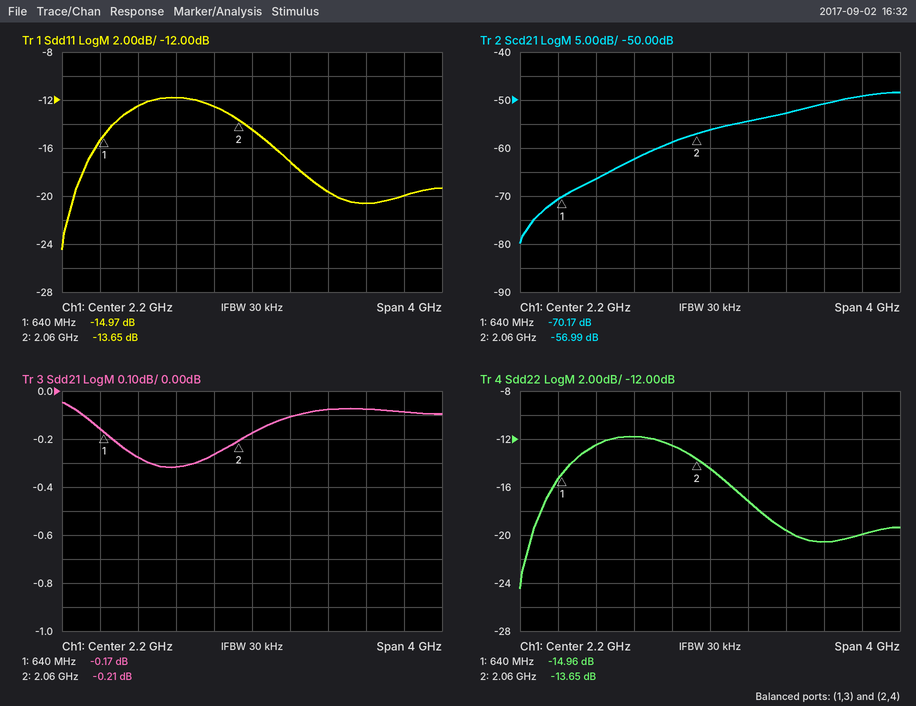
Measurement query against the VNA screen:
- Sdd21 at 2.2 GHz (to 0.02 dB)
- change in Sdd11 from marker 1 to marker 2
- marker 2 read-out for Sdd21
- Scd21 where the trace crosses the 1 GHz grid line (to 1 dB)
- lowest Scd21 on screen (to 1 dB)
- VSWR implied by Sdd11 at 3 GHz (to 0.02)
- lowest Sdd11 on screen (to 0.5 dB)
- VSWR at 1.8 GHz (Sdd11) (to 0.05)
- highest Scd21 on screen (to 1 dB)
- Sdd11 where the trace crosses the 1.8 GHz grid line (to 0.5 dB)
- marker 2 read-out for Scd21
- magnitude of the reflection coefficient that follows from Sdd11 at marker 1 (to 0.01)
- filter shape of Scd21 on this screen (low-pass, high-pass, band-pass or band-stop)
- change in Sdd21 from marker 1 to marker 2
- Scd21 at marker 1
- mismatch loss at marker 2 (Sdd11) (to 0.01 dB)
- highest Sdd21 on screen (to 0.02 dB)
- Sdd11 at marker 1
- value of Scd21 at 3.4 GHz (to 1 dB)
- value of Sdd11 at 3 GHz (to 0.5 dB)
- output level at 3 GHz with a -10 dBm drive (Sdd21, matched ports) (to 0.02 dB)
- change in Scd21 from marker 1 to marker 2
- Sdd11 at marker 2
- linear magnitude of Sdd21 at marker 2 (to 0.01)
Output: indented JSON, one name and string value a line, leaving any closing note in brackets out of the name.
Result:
{
  "Sdd21 at 2.2 GHz": "-0.18 dB",
  "change in Sdd11 from marker 1 to marker 2": "1.32 dB",
  "marker 2 read-out for Sdd21": "-0.21 dB",
  "Scd21 where the trace crosses the 1 GHz grid line": "-66 dB",
  "lowest Scd21 on screen": "-80 dB",
  "VSWR implied by Sdd11 at 3 GHz": "1.24",
  "lowest Sdd11 on screen": "-24.5 dB",
  "VSWR at 1.8 GHz (Sdd11)": "1.60",
  "highest Scd21 on screen": "-48 dB",
  "Sdd11 where the trace crosses the 1.8 GHz grid line": "-12.5 dB",
  "marker 2 read-out for Scd21": "-56.99 dB",
  "magnitude of the reflection coefficient that follows from Sdd11 at marker 1": "0.18",
  "filter shape of Scd21 on this screen": "high-pass",
  "change in Sdd21 from marker 1 to marker 2": "-0.04 dB",
  "Scd21 at marker 1": "-70.17 dB",
  "mismatch loss at marker 2 (Sdd11)": "0.19 dB",
  "highest Sdd21 on screen": "-0.04 dB",
  "Sdd11 at marker 1": "-14.97 dB",
  "value of Scd21 at 3.4 GHz": "-51 dB",
  "value of Sdd11 at 3 GHz": "-19.5 dB",
  "output level at 3 GHz with a -10 dBm drive (Sdd21, matched ports)": "-10.08 dBm",
  "change in Scd21 from marker 1 to marker 2": "13.18 dB",
  "Sdd11 at marker 2": "-13.65 dB",
  "linear magnitude of Sdd21 at marker 2": "0.98"
}
